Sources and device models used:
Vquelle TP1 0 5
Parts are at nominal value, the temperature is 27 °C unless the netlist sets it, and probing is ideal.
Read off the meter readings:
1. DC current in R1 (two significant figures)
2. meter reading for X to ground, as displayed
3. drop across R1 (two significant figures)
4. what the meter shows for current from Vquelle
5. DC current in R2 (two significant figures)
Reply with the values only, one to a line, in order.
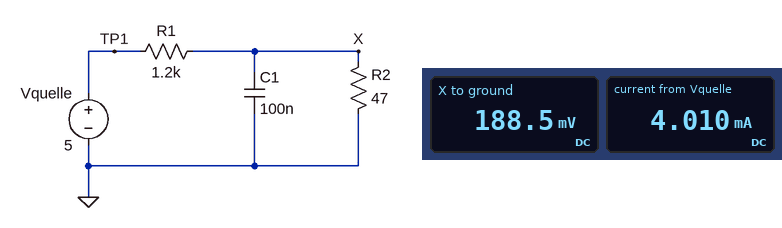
4.0 mA
188.5 mV
4.8 V
4.010 mA
4.0 mA
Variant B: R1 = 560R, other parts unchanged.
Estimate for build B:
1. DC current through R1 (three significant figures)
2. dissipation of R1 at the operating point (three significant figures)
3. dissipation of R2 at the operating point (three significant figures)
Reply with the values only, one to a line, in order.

8.24 mA
38.0 mW
3.19 mW
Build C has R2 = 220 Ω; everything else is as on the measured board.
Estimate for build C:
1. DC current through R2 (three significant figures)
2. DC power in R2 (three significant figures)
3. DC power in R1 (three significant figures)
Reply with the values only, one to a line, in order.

3.52 mA
2.73 mW
14.9 mW
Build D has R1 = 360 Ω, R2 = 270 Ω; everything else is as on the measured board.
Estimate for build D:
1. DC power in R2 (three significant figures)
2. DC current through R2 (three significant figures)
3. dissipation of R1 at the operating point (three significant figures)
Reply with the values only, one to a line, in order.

17.0 mW
7.94 mA
22.7 mW
